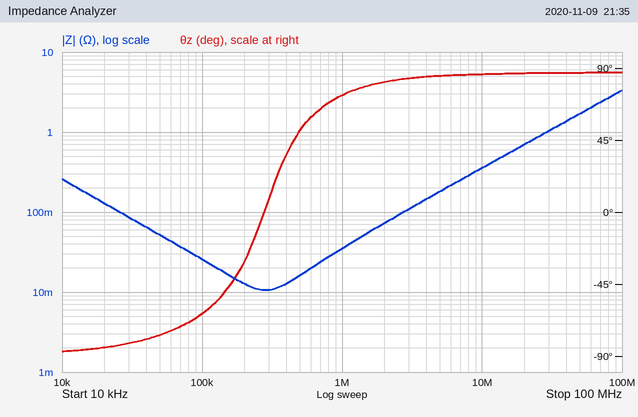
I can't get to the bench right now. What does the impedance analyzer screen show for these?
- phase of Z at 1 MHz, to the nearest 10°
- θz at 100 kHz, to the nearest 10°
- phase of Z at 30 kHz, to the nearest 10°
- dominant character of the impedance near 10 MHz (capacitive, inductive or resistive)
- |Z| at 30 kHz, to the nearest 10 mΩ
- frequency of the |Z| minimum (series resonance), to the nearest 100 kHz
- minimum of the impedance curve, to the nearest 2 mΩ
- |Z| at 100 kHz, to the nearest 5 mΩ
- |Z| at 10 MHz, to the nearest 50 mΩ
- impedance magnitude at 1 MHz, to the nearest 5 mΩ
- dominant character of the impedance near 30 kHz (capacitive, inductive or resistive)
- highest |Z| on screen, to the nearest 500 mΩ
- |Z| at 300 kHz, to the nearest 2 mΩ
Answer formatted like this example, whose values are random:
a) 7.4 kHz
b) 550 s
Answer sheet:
a) 70°
b) -60°
c) -80°
d) inductive
e) 90 mΩ
f) 300 kHz
g) 10 mΩ
h) 25 mΩ
i) 350 mΩ
j) 35 mΩ
k) capacitive
l) 3.5 Ω
m) 10 mΩ
